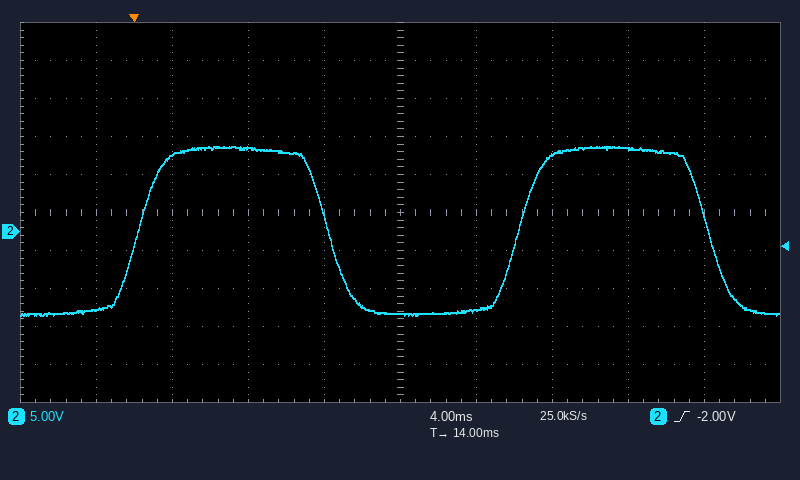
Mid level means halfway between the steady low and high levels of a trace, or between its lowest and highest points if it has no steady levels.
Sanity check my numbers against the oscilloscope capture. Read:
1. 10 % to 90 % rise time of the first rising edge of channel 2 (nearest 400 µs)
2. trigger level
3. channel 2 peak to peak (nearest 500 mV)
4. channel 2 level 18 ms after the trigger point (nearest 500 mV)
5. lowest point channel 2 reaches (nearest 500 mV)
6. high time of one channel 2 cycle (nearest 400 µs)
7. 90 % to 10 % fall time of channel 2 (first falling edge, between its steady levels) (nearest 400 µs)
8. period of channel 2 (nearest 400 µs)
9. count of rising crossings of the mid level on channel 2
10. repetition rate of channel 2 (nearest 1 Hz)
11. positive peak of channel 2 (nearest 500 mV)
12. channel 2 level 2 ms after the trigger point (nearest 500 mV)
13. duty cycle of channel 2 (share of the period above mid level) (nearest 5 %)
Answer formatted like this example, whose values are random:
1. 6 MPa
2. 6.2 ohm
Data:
1. 2.4 ms
2. -2.00 V
3. 22.0 V
4. -10.5 V
5. -11.0 V
6. 10.0 ms
7. 2.4 ms
8. 20.0 ms
9. 2
10. 50 Hz
11. 11.0 V
12. 10.0 V
13. 50 %
